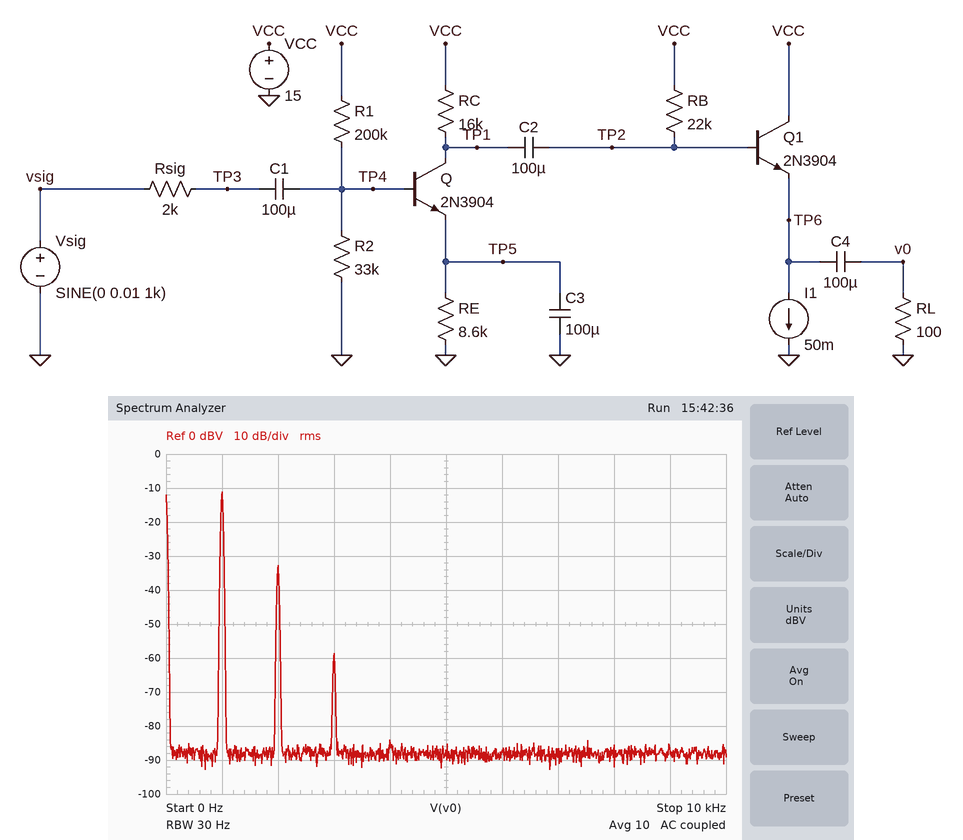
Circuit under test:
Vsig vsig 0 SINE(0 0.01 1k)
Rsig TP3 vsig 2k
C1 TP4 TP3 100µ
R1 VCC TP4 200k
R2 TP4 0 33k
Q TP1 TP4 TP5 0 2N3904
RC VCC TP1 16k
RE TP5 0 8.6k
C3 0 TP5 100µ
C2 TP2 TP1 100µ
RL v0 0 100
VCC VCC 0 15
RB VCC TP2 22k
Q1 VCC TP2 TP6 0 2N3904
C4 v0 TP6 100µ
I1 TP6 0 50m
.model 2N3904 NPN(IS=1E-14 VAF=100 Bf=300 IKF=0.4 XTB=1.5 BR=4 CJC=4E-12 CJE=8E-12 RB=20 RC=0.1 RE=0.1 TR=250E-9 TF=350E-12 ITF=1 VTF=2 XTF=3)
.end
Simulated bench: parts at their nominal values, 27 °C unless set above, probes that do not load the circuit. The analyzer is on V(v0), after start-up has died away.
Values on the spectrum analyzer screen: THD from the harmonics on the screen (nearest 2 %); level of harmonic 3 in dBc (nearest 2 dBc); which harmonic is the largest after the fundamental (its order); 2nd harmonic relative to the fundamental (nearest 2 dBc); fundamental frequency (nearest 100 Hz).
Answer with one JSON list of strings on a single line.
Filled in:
["8 %", "-48 dBc", "2", "-22 dBc", "1.0 kHz"]
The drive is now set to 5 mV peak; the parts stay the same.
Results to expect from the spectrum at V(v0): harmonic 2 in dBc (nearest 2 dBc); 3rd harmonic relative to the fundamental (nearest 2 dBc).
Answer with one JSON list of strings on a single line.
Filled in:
["-28 dBc", "-60 dBc"]
